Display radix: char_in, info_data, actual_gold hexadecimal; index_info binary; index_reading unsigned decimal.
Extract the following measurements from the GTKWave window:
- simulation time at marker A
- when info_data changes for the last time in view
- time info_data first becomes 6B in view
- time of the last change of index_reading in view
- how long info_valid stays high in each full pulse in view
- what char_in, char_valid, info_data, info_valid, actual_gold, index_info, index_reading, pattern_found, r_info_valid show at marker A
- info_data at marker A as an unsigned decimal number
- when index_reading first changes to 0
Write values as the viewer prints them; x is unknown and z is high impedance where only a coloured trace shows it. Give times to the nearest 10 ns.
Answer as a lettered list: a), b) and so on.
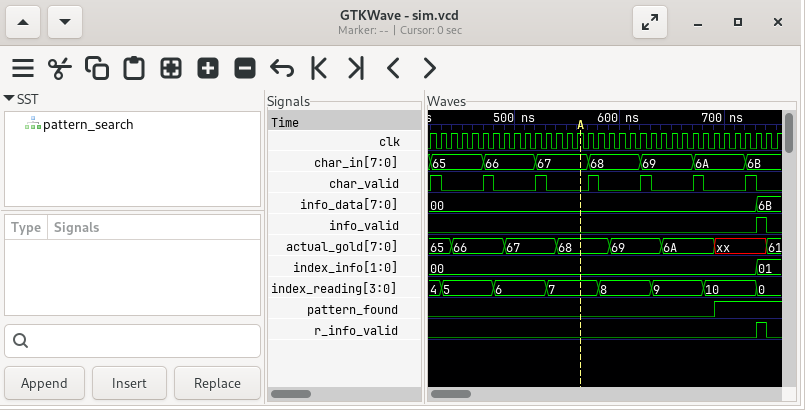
a) 560 ns
b) 730 ns
c) 730 ns
d) 730 ns
e) 10 ns
f) char_in=67, char_valid=0, info_data=00, info_valid=0, actual_gold=68, index_info=00, index_reading=7, pattern_found=0, r_info_valid=0
g) 0
h) 730 ns
